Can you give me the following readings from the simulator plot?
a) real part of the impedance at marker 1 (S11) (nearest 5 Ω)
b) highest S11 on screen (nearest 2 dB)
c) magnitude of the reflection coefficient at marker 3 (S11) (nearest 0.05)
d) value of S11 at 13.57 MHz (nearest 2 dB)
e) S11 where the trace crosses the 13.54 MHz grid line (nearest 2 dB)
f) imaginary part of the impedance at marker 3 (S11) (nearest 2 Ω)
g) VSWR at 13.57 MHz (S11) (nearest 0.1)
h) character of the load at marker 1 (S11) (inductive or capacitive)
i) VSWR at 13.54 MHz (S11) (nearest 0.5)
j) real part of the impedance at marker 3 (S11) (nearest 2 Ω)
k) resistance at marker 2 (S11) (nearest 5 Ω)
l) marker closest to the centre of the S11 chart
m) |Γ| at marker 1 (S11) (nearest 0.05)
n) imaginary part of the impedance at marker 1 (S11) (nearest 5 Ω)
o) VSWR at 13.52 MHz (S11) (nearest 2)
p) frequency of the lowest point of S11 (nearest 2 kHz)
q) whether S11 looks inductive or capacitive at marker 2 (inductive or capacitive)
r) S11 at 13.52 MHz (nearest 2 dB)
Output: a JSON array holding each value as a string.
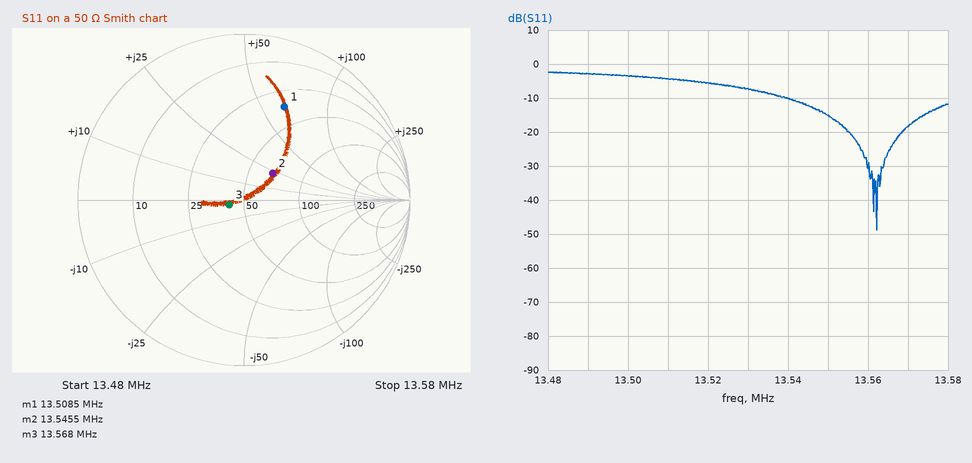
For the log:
["35 Ω", "-2 dB", "0.10", "-18 dB", "-10 dB", "-2 Ω", "1.3", "inductive", "2.0", "42 Ω", "65 Ω", "marker 3", "0.60", "+65 Ω", "4", "13.562 MHz", "inductive", "-6 dB"]
